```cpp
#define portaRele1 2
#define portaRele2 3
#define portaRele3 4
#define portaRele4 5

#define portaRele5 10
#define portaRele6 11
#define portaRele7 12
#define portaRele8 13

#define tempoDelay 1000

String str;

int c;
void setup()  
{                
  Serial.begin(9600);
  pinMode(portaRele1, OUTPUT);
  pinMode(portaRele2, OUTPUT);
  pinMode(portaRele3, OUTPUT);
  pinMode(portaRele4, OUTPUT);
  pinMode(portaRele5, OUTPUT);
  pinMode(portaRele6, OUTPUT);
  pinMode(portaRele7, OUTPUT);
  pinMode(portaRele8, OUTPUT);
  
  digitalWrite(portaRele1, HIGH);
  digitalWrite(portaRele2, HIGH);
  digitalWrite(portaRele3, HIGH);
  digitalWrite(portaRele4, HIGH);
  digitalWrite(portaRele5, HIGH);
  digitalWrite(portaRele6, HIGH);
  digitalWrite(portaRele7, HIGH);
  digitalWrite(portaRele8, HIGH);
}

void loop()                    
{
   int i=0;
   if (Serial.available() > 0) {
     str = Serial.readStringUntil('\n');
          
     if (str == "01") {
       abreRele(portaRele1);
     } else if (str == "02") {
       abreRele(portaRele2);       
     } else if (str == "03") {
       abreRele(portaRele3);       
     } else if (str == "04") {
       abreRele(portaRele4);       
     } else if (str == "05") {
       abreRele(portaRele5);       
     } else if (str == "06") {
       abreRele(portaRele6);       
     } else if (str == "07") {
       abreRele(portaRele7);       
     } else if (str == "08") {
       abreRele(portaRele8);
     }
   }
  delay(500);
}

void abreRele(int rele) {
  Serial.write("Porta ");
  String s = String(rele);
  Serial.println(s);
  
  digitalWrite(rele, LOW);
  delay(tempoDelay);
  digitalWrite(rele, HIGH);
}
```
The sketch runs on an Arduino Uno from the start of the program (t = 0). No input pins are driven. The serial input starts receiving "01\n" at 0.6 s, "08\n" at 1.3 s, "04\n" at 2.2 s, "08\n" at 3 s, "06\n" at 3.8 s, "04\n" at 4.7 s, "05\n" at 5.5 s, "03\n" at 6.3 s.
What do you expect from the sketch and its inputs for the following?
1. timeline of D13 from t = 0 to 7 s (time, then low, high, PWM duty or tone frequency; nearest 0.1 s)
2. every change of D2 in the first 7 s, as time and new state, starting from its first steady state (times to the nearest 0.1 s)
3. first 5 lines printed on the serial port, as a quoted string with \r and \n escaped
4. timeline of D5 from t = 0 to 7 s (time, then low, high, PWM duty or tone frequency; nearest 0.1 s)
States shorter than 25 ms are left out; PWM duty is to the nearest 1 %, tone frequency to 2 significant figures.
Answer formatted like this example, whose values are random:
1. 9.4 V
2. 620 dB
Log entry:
1. 0 s high; 2.5 s low; 3.5 s high; 5.5 s low; 6.5 s high
2. 0 s high; 1 s low; 2 s high
3. "Porta 2\r\nPorta 13\r\nPorta 5\r\nPorta 13\r\nPorta 11\r\n"
4. 0 s high; 4 s low; 5 s high
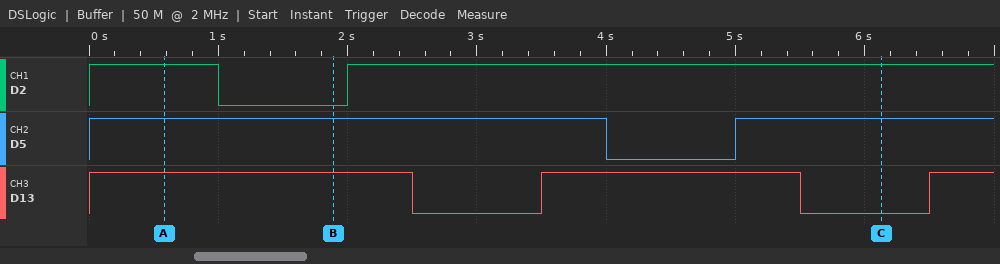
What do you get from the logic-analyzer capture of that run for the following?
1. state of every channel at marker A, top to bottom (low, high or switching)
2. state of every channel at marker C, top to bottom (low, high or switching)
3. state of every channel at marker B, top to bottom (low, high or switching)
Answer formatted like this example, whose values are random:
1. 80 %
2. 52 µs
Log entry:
1. D2 high, D5 high, D13 high
2. D2 high, D5 high, D13 low
3. D2 low, D5 high, D13 high
